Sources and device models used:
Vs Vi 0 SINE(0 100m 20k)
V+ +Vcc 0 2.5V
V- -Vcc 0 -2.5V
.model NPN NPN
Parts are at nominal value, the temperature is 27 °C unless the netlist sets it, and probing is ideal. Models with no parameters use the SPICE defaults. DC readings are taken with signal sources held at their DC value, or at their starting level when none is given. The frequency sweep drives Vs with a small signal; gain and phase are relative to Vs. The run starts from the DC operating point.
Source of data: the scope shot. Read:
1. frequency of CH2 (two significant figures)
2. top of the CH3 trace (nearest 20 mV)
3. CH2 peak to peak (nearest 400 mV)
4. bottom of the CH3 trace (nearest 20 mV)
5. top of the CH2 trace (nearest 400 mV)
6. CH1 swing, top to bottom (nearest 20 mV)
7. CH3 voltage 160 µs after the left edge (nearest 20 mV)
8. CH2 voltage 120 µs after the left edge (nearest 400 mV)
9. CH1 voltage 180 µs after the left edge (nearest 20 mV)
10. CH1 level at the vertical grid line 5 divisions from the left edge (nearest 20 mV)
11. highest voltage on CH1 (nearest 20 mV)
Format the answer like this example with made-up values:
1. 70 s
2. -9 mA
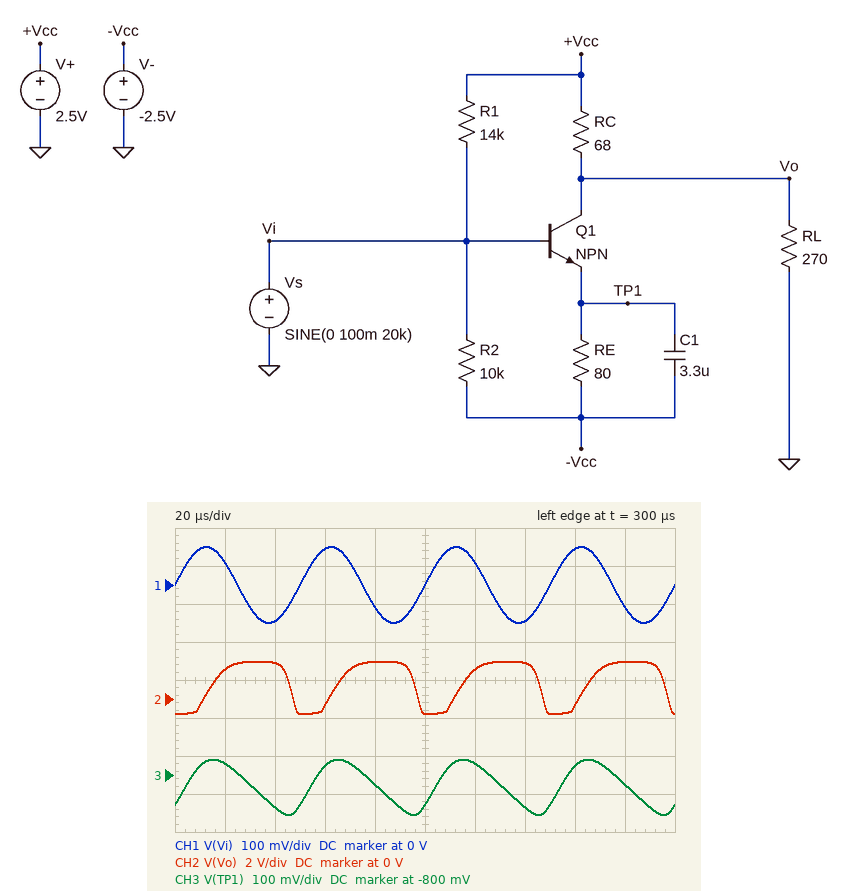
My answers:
1. 20 kHz
2. -760 mV
3. 2.8 V
4. -900 mV
5. 2.0 V
6. 200 mV
7. -780 mV
8. 1.6 V
9. -60 mV
10. 0 V
11. 100 mV
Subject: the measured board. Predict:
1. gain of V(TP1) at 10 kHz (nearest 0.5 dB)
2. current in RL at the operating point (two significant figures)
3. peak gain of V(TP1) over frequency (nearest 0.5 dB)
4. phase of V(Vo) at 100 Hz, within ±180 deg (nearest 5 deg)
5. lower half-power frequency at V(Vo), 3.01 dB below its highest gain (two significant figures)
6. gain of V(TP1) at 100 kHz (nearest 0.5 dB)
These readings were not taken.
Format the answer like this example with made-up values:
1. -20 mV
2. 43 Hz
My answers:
1. -0.5 dB
2. 3.3 mA
3. 0 dB
4. -170 deg
5. 39 kHz
6. -9.0 dB
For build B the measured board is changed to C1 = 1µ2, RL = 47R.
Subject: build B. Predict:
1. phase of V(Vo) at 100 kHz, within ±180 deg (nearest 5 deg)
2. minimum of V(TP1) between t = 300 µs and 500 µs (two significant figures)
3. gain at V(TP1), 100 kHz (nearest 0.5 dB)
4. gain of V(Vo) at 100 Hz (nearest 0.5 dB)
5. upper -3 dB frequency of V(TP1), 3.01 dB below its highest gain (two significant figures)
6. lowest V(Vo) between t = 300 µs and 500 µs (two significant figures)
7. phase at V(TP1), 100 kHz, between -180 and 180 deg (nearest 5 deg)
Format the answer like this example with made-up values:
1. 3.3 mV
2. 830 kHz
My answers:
1. -135 deg
2. -950 mV
3. -3.0 dB
4. -9.5 dB
5. 110 kHz
6. 46 mV
7. -45 deg
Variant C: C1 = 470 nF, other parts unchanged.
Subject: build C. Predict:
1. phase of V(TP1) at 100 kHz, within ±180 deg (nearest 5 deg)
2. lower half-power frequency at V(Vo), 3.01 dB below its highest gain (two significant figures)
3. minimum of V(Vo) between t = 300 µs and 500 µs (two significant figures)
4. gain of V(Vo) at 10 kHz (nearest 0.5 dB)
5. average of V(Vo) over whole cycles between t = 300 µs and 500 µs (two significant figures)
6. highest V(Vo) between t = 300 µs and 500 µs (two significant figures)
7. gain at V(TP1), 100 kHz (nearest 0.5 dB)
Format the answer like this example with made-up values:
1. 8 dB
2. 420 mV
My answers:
1. -20 deg
2. 270 kHz
3. 570 mV
4. 4.5 dB
5. 890 mV
6. 1.2 V
7. -0.5 dB
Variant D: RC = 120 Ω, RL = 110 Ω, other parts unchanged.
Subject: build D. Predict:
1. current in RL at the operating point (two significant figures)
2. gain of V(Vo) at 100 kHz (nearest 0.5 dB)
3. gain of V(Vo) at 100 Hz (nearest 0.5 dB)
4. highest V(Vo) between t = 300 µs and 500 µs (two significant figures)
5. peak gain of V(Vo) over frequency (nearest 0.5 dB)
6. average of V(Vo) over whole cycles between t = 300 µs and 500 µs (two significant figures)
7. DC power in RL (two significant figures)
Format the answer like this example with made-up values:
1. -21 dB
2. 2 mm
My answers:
1. 230 µA
2. 32.5 dB
3. -3.0 dB
4. 1.2 V
5. 33.0 dB
6. 270 mV
7. 5.8 µW
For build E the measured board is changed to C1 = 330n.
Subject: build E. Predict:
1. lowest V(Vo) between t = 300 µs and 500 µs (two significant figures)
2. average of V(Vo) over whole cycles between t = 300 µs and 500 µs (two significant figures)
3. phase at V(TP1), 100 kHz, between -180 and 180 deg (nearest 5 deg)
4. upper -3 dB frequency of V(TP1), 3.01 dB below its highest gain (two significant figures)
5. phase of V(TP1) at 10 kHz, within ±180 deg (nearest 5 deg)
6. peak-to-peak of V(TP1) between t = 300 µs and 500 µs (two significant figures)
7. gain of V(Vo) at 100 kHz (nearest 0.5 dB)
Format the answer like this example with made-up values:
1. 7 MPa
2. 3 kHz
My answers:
1. 660 mV
2. 890 mV
3. -15 deg
4. 390 kHz
5. 0 deg
6. 200 mV
7. 20.5 dB
